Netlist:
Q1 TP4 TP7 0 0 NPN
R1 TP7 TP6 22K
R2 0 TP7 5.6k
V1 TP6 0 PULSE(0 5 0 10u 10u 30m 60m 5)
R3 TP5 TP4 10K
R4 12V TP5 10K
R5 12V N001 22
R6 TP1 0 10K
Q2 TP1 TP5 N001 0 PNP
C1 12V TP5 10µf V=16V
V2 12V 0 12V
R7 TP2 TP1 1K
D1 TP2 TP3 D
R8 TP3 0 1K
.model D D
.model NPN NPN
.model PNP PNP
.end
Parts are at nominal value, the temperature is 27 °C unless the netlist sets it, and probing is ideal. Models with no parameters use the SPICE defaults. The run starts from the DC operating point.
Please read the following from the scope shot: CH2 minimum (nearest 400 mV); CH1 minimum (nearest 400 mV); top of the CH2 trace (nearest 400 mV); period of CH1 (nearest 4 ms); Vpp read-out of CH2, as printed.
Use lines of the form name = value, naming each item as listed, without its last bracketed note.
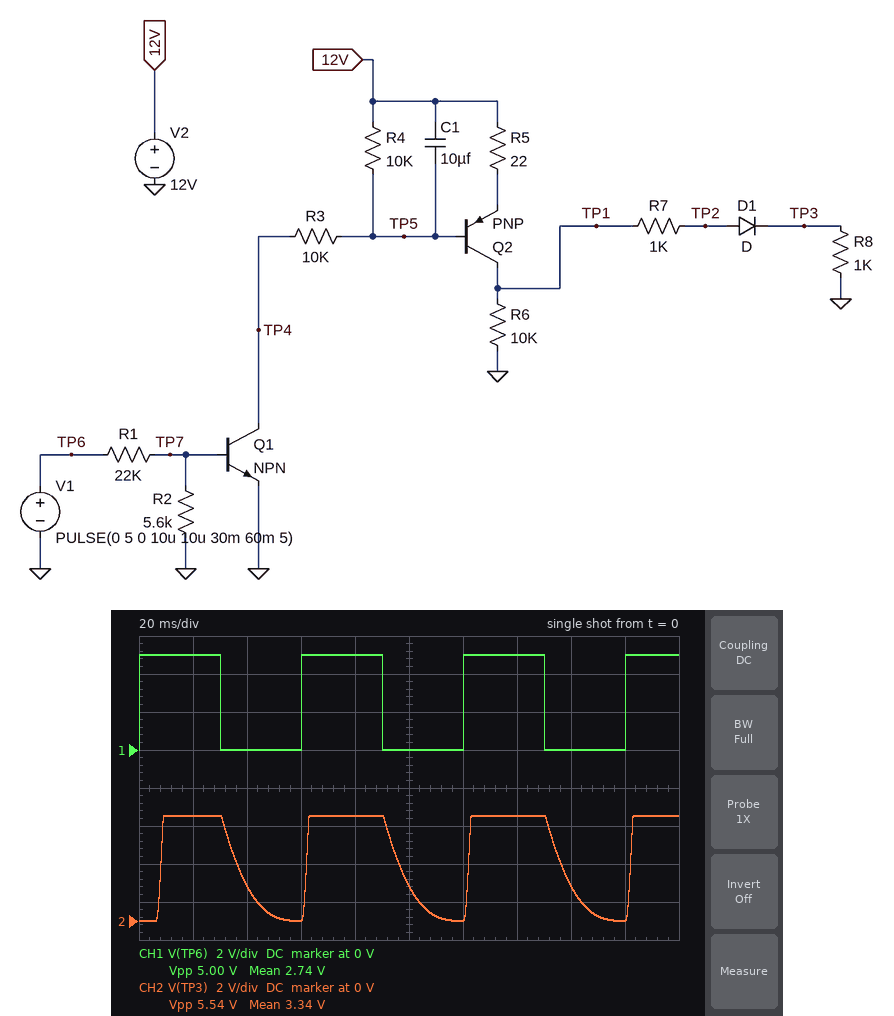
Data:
CH2 minimum = 0 V
CH1 minimum = 0 V
top of the CH2 trace = 5.6 V
period of CH1 = 60 ms
Vpp read-out of CH2, as printed = 5.54 V
